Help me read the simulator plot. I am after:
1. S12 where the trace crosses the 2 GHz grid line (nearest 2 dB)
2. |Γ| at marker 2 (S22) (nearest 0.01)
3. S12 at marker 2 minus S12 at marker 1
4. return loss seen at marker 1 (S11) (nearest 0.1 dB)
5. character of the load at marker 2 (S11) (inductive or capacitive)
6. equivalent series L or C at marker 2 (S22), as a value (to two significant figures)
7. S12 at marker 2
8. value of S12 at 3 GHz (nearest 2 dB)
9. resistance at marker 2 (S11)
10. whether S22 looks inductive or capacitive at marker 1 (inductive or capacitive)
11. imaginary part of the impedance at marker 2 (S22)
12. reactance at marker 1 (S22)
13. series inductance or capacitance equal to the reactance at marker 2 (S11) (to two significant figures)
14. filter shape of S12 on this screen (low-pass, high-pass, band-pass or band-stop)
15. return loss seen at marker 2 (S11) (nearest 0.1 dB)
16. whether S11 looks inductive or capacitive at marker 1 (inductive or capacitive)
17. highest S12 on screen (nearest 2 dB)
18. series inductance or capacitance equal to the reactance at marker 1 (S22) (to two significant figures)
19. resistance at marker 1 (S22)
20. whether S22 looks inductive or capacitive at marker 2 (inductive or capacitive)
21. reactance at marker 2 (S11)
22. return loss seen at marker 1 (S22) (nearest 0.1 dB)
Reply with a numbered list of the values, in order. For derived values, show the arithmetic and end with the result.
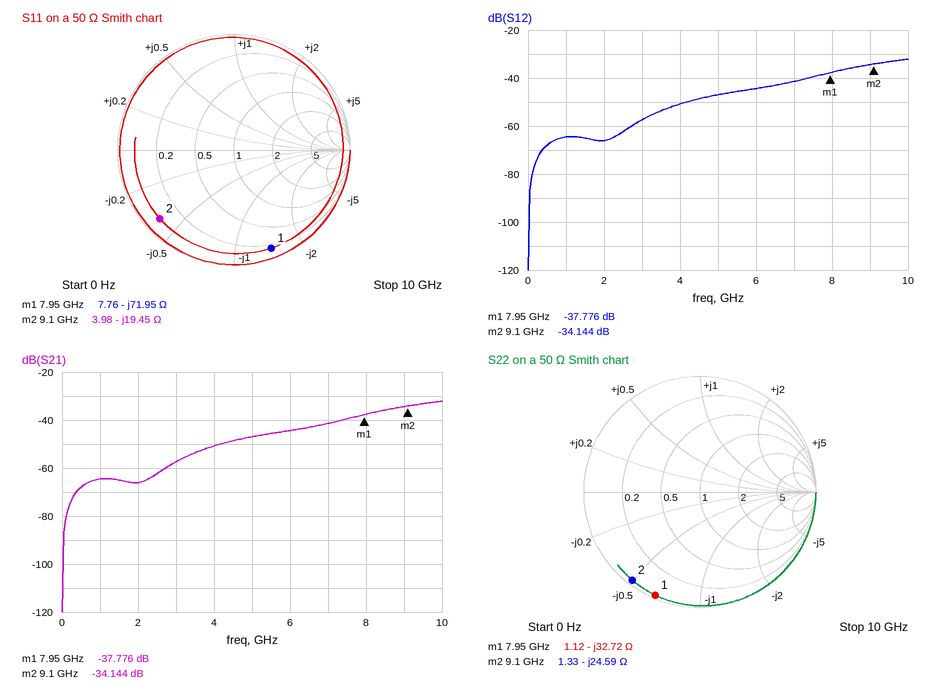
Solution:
1. -66 dB
2. 0.96
3. -34.144 − (-37.776) = 3.632 dB
4. 0.9 dB
5. capacitive
6. C = 1/(2π × 9.1 GHz × 24.59 Ω) ≈ 711 fF, so 710 fF to two significant figures
7. -34.144 dB
8. -58 dB
9. 3.98 Ω
10. capacitive
11. -24.59 Ω
12. -32.72 Ω
13. C = 1/(2π × 9.1 GHz × 19.45 Ω) ≈ 899 fF, so 900 fF to two significant figures
14. high-pass
15. 1.2 dB
16. capacitive
17. -32 dB
18. C = 1/(2π × 7.95 GHz × 32.72 Ω) ≈ 612 fF, so 610 fF to two significant figures
19. 1.12 Ω
20. capacitive
21. -19.45 Ω
22. 0.3 dB
